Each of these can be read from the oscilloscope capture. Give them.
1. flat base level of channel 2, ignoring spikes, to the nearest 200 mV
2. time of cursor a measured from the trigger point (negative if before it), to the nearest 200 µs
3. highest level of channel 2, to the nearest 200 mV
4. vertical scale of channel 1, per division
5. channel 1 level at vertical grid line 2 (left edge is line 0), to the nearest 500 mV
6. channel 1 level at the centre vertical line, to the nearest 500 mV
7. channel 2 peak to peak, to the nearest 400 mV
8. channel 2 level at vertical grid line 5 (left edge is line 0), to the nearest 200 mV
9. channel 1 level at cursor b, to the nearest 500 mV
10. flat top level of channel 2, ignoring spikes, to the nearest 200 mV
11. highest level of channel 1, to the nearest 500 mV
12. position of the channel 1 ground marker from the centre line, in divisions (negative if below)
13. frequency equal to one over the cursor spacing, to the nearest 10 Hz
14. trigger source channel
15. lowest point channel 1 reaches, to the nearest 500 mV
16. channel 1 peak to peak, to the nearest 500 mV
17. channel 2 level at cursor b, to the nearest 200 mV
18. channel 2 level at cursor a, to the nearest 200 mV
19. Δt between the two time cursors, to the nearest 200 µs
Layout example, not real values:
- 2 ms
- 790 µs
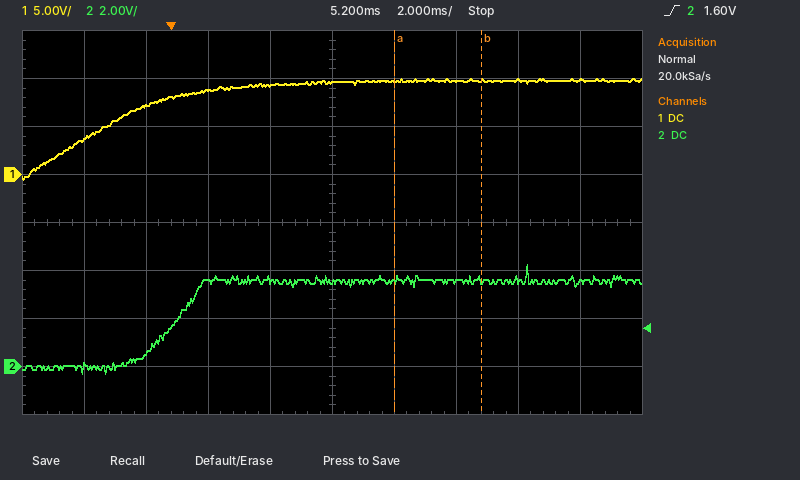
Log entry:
- 0.0 V
- +7.2 ms
- 4.2 V
- 5 V
- 7.0 V
- 9.5 V
- 4.4 V
- 3.6 V
- 10.0 V
- 3.6 V
- 10.0 V
- +1.0 div
- 360 Hz
- channel 2
- -500 mV
- 10.5 V
- 3.6 V
- 3.6 V
- 2.8 ms
